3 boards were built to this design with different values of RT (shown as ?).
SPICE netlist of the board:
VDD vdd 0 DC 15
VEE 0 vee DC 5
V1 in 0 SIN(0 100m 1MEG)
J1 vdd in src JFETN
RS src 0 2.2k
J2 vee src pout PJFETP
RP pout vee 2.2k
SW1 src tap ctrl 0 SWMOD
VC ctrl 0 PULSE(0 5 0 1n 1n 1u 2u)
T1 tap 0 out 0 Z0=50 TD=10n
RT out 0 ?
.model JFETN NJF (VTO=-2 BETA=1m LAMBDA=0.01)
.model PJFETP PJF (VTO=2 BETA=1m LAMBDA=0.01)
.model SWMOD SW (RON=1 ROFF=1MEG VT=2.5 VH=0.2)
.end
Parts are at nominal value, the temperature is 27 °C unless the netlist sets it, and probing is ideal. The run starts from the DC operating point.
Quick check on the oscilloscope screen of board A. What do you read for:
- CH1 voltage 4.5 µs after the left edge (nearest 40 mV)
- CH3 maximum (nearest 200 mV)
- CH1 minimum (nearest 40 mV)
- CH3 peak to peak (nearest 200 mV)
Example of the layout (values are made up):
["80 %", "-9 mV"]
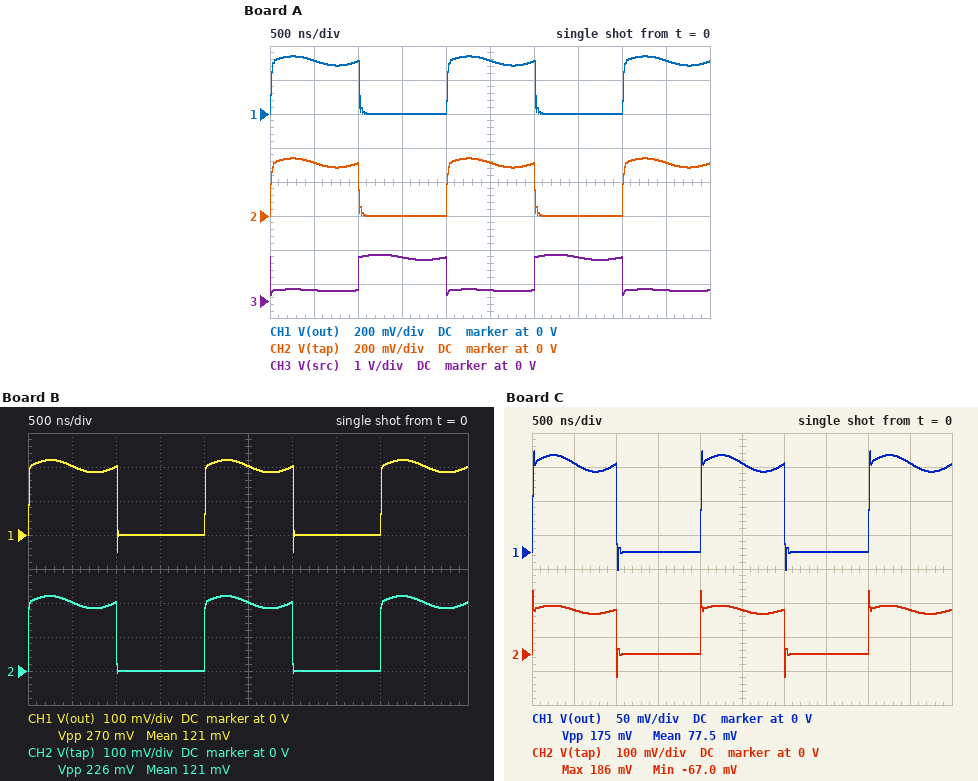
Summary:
["320 mV", "1.4 V", "0 V", "1.2 V"]
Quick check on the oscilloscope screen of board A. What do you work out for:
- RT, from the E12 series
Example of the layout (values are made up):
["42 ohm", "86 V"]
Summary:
["100 Ω"]
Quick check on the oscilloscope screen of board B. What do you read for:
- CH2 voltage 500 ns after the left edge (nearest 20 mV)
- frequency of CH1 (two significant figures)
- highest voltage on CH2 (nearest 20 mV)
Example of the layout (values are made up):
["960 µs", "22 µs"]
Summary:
["200 mV", "500 kHz", "220 mV"]
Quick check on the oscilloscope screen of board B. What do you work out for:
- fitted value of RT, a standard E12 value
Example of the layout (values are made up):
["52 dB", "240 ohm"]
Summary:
["56 Ω"]
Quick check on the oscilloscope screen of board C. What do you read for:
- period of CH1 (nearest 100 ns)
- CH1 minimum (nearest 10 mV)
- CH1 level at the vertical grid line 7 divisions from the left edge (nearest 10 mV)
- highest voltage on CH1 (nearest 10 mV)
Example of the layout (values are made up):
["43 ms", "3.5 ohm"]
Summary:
["2.0 µs", "-30 mV", "0 V", "150 mV"]
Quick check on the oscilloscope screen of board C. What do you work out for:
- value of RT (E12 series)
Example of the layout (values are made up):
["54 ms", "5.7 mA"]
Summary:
["33 Ω"]
